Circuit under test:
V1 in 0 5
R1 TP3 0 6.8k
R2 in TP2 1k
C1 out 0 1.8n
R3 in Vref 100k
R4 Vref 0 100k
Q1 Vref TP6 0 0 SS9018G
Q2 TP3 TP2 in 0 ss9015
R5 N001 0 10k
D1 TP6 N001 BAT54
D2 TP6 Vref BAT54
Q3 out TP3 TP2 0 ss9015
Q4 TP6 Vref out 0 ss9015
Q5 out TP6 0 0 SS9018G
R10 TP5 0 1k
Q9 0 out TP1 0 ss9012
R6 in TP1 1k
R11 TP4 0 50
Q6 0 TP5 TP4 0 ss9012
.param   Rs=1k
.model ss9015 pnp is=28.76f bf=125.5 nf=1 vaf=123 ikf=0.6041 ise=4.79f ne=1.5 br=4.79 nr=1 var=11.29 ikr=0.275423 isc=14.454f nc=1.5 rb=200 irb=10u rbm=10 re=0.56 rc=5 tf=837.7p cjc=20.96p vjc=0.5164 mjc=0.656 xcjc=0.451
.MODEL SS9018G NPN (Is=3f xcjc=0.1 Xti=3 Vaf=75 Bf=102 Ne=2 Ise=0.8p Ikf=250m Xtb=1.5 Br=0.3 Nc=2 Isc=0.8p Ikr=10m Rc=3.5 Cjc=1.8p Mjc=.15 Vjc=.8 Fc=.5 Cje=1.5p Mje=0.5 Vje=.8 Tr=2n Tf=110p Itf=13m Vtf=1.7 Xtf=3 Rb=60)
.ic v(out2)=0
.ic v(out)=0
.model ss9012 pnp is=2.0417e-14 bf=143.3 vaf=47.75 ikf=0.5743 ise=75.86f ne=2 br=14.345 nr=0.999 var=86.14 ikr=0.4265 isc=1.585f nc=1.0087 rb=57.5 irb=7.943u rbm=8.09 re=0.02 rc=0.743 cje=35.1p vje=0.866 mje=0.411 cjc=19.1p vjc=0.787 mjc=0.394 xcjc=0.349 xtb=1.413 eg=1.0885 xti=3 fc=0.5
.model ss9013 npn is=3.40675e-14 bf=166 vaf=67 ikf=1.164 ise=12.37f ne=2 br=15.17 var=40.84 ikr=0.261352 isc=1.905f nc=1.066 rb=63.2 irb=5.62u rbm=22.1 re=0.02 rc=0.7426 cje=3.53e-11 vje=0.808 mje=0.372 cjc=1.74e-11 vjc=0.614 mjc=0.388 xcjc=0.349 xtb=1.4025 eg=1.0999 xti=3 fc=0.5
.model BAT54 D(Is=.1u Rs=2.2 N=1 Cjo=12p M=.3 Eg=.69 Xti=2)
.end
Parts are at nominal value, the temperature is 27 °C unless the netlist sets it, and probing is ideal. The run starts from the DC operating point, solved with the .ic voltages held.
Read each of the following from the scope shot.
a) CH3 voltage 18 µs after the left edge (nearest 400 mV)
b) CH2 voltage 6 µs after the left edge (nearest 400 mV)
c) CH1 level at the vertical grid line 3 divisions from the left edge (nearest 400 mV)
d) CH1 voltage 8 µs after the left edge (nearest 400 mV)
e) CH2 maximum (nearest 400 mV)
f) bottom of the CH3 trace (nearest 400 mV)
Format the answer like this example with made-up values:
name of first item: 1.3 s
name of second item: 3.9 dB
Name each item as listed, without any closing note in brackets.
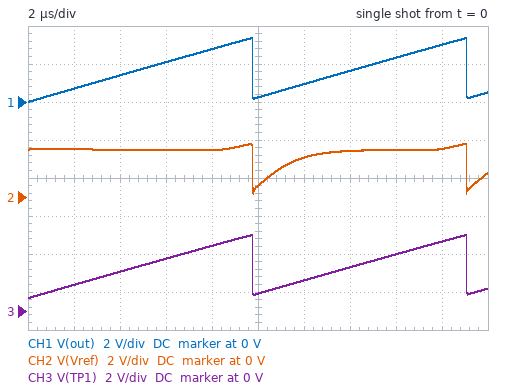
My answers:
CH3 voltage 18 µs after the left edge: 3.6 V
CH2 voltage 6 µs after the left edge: 2.4 V
CH1 level at the vertical grid line 3 divisions from the left edge: 2.0 V
CH1 voltage 8 µs after the left edge: 2.8 V
CH2 maximum: 2.8 V
bottom of the CH3 trace: 800 mV
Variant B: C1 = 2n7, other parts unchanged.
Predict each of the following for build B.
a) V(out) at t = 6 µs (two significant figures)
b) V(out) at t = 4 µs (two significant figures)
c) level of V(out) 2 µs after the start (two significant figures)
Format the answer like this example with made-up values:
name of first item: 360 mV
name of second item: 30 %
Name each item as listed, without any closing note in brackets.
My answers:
V(out) at t = 6 µs: 1.4 V
V(out) at t = 4 µs: 940 mV
level of V(out) 2 µs after the start: 470 mV
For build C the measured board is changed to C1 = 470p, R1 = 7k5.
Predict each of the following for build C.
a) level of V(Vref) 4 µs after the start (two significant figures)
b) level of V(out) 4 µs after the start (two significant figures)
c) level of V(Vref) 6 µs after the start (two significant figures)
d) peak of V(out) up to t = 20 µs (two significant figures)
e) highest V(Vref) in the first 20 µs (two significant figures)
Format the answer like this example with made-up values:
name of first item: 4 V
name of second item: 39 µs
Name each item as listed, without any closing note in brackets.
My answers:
level of V(Vref) 4 µs after the start: 1.5 V
level of V(out) 4 µs after the start: 1.7 V
level of V(Vref) 6 µs after the start: 1.3 V
peak of V(out) up to t = 20 µs: 3.5 V
highest V(Vref) in the first 20 µs: 2.9 V
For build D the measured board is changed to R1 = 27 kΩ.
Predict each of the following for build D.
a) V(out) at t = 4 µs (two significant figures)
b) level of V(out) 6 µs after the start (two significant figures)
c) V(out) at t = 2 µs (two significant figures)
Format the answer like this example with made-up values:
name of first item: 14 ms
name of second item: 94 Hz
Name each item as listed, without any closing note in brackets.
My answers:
V(out) at t = 4 µs: 1.3 V
level of V(out) 6 µs after the start: 2.0 V
V(out) at t = 2 µs: 660 mV
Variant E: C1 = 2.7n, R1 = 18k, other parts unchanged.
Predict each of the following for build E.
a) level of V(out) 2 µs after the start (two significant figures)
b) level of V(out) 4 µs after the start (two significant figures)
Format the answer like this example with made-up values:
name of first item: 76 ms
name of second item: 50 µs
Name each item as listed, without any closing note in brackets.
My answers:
level of V(out) 2 µs after the start: 450 mV
level of V(out) 4 µs after the start: 900 mV
